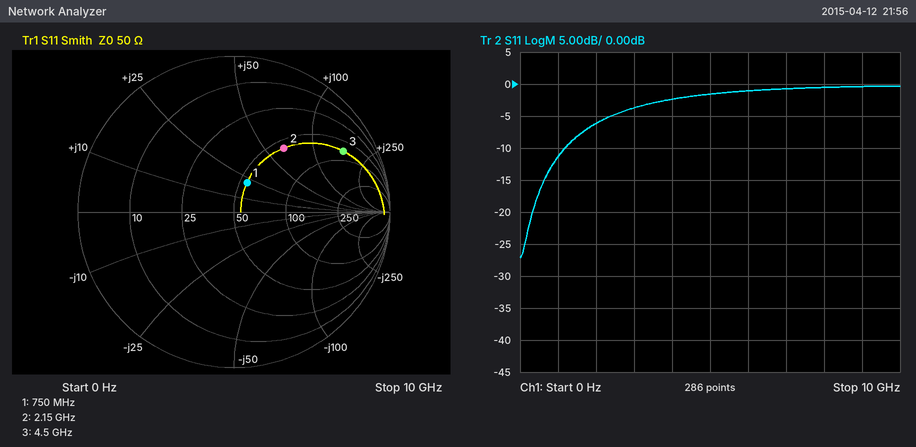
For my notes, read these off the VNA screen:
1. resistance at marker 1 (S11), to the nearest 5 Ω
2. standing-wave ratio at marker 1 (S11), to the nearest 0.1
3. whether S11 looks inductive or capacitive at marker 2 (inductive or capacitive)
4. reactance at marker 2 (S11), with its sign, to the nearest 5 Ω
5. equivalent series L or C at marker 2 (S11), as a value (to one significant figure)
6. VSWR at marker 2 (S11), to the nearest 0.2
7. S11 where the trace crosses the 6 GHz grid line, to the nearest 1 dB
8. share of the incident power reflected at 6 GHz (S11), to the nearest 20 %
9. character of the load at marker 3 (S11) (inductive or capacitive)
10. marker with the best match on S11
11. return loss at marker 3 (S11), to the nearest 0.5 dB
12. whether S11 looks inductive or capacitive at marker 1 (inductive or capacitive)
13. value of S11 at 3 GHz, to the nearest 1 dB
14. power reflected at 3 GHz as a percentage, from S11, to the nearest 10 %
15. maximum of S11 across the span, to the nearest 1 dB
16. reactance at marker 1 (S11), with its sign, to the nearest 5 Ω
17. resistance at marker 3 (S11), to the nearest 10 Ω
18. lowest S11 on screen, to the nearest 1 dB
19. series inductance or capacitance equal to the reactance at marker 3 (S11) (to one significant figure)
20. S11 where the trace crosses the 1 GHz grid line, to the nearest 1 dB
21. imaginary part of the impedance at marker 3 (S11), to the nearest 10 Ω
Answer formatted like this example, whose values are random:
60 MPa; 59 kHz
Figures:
55 Ω; 1.5; inductive; +65 Ω; 5 nH; 3.2; -1 dB; 80 %; inductive; marker 1; 2.0 dB; inductive; -4 dB; 40 %; 0 dB; +20 Ω; 70 Ω; -27 dB; 6 nH; -11 dB; +160 Ω
